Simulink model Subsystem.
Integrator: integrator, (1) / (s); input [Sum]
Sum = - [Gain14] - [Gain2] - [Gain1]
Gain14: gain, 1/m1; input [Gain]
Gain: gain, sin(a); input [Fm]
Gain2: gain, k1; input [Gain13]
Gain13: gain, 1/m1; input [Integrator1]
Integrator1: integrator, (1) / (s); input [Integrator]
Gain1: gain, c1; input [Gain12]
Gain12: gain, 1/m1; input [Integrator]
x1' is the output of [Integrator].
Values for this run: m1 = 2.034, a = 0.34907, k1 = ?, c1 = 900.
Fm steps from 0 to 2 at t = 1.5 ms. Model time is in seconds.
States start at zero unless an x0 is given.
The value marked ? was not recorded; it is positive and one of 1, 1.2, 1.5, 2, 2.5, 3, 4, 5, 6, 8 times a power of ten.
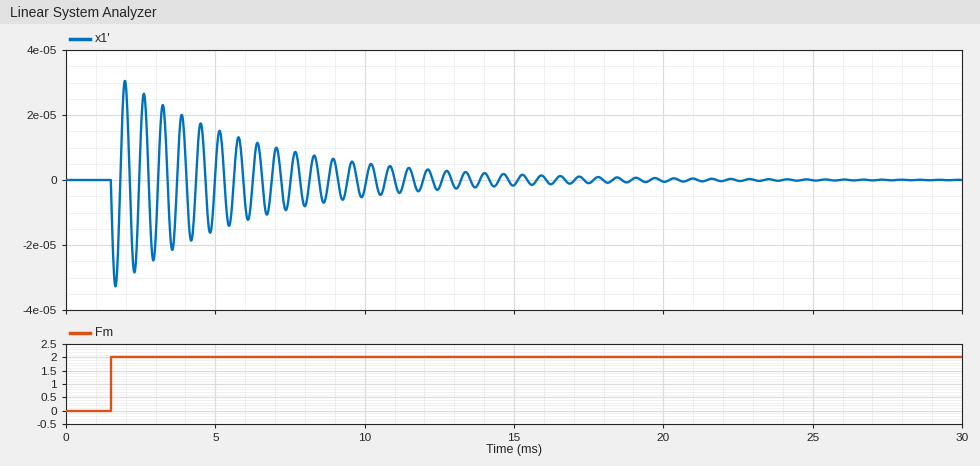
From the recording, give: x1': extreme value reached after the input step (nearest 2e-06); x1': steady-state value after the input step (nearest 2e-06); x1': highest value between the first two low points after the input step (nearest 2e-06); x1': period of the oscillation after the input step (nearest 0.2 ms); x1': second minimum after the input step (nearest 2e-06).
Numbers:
-0.000032
0.000000
0.000030
0.6 ms
-0.000028
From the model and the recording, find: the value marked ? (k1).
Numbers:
2e+08
